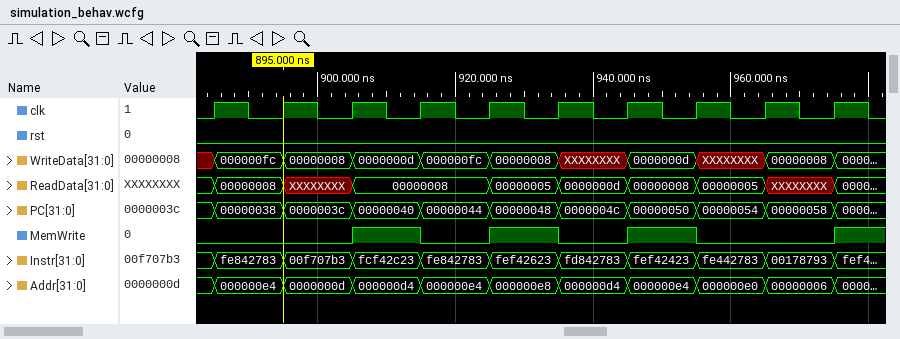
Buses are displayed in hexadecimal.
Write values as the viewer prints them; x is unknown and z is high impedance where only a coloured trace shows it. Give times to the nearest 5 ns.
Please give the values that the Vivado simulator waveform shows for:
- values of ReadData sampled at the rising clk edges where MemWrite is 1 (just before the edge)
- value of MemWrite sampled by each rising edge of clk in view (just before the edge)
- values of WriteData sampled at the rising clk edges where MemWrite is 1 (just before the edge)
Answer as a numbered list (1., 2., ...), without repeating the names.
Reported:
1. 00000008, 00000005, 00000008
2. 0 0 0 1 0 1 0 1 0 0
3. 0000000d, 00000008, 0000000d
